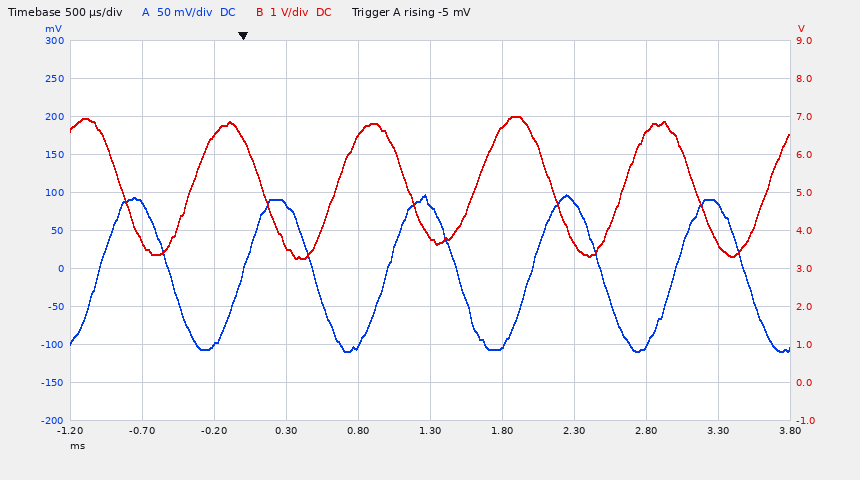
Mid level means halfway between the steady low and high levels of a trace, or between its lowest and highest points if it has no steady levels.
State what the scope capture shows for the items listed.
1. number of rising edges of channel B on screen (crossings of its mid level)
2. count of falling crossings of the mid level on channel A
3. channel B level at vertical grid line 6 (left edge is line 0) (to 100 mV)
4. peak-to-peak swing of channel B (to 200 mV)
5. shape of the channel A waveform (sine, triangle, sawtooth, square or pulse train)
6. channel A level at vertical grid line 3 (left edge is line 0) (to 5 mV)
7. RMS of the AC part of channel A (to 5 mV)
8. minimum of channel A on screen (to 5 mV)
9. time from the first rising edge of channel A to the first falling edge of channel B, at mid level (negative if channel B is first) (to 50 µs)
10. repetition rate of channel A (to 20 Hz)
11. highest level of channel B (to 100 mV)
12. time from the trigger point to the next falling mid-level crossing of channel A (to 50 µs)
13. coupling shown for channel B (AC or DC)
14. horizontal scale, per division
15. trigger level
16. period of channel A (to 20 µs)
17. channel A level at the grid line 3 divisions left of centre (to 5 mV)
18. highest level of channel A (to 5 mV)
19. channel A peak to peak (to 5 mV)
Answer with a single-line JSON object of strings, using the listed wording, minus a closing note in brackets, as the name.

{"number of rising edges of channel B on screen": "5", "count of falling crossings of the mid level on channel A": "5", "channel B level at vertical grid line 6 (left edge is line 0)": "6.7 V", "peak-to-peak swing of channel B": "3.8 V", "shape of the channel A waveform": "sine", "channel A level at vertical grid line 3 (left edge is line 0)": "85 mV", "RMS of the AC part of channel A": "70 mV", "minimum of channel A on screen": "-110 mV", "time from the first rising edge of channel A to the first falling edge of channel B, at mid level (negative if channel B is first)": "+150 µs", "repetition rate of channel A": "1.00 kHz", "highest level of channel B": "7.0 V", "time from the trigger point to the next falling mid-level crossing of channel A": "500 µs", "coupling shown for channel B": "DC", "horizontal scale, per division": "500 µs", "trigger level": "-5 mV", "period of channel A": "1.00 ms", "channel A level at the grid line 3 divisions left of centre": "-100 mV", "highest level of channel A": "95 mV", "channel A peak to peak": "205 mV"}
